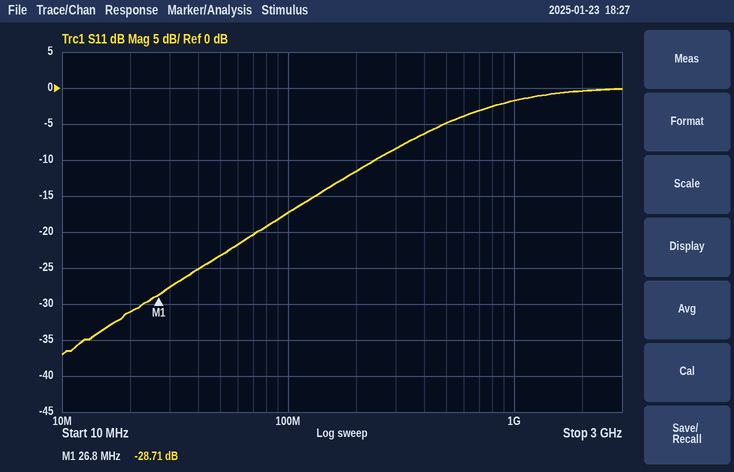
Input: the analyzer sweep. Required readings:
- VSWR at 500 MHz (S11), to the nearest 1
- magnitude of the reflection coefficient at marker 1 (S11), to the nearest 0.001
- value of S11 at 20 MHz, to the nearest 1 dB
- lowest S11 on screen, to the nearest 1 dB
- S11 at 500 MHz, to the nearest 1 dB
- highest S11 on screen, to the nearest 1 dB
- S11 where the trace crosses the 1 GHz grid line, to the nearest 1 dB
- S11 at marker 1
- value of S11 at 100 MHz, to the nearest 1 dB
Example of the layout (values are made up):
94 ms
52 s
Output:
4
0.037
-31 dB
-37 dB
-5 dB
0 dB
-2 dB
-28.71 dB
-17 dB
